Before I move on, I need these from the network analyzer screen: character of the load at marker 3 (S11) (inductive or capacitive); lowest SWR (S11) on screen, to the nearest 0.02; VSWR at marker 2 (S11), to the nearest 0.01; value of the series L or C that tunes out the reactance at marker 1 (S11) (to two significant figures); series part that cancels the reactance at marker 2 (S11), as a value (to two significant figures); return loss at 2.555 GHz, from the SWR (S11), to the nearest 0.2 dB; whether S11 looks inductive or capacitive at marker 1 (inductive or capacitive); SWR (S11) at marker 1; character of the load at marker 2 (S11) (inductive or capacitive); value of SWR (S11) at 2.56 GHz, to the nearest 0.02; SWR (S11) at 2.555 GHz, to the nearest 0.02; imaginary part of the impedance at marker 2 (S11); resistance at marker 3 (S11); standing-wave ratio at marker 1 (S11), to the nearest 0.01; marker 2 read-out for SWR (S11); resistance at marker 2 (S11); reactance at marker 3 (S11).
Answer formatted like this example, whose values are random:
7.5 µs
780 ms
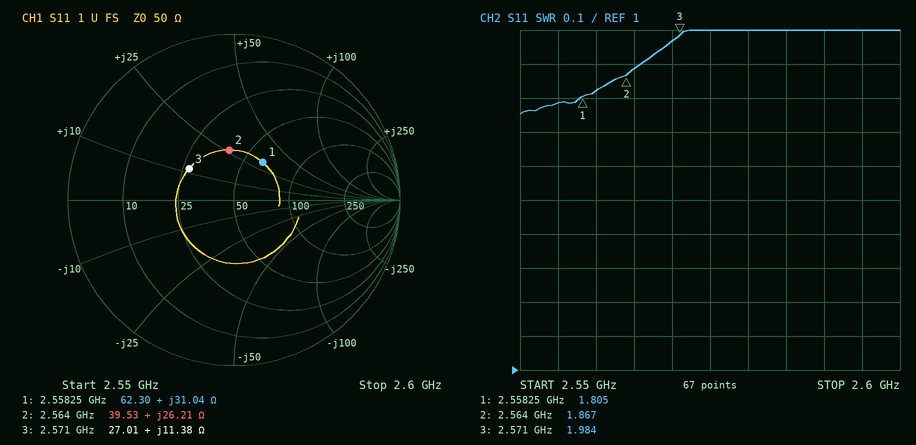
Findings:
inductive
1.76
1.87
2.0 pF
2.4 pF
11.0 dB
inductive
1.805
inductive
1.82
1.78
+26.21 Ω
27.01 Ω
1.80
1.867
39.53 Ω
+11.38 Ω
